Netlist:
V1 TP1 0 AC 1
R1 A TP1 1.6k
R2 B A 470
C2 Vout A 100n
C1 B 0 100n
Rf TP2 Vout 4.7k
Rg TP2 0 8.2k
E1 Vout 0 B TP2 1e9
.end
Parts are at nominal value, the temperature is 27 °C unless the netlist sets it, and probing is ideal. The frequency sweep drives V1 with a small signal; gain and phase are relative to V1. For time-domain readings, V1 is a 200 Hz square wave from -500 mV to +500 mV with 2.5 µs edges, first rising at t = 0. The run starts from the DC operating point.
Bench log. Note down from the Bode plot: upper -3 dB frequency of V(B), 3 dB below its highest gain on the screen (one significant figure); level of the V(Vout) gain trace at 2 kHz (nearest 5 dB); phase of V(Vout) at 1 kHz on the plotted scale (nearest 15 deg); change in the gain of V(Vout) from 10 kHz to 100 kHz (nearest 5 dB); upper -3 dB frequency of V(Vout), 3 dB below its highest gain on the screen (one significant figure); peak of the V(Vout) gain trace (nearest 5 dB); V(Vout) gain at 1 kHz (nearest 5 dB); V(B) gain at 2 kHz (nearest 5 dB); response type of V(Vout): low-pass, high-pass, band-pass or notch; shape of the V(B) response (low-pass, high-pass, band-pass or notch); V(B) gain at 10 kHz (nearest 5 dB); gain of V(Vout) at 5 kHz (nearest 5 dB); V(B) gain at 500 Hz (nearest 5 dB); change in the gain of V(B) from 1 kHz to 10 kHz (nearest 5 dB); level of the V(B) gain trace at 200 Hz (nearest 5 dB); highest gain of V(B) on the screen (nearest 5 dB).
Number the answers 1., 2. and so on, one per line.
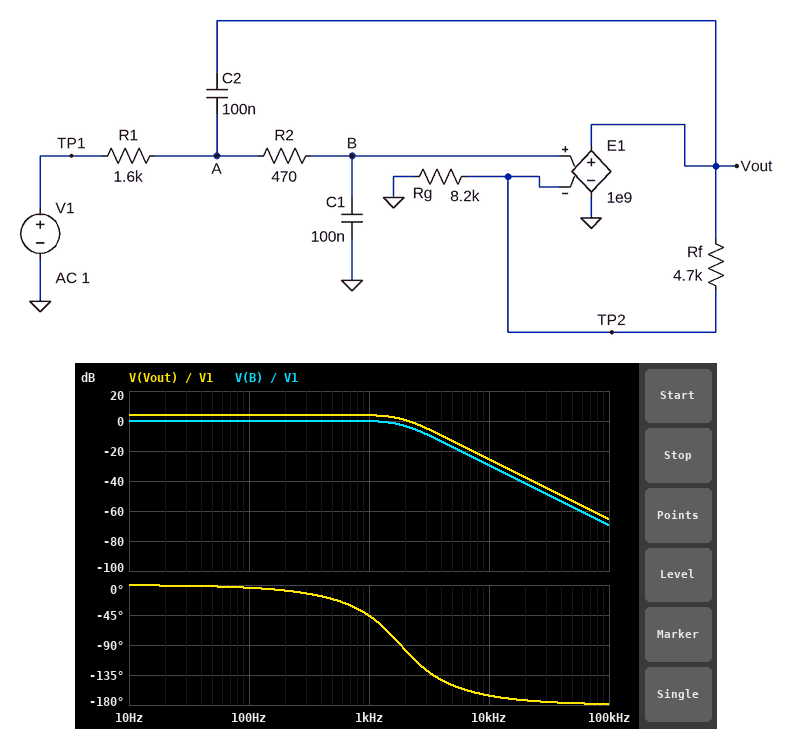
1. 2 kHz
2. 0 dB
3. -45 deg
4. -40 dB
5. 2 kHz
6. 5 dB
7. 5 dB
8. -5 dB
9. low-pass
10. low-pass
11. -30 dB
12. -15 dB
13. 0 dB
14. -30 dB
15. 0 dB
16. 0 dB
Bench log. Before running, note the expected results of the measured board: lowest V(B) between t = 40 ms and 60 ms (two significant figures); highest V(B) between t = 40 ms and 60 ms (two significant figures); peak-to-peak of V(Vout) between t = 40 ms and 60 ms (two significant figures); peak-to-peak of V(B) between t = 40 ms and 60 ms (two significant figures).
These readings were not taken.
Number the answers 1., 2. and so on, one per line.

1. -560 mV
2. 560 mV
3. 1.8 V
4. 1.1 V
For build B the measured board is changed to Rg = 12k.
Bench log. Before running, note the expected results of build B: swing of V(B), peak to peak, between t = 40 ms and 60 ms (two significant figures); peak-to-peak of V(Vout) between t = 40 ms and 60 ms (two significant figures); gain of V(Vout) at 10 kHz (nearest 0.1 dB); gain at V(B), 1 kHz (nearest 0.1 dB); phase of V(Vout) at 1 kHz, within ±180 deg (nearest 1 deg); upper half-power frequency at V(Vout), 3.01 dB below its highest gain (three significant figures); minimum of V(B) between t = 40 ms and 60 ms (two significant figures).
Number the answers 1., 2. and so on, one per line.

1. 1.0 V
2. 1.4 V
3. -26.7 dB
4. -1.2 dB
5. -52 deg
6. 1.52 kHz
7. -510 mV
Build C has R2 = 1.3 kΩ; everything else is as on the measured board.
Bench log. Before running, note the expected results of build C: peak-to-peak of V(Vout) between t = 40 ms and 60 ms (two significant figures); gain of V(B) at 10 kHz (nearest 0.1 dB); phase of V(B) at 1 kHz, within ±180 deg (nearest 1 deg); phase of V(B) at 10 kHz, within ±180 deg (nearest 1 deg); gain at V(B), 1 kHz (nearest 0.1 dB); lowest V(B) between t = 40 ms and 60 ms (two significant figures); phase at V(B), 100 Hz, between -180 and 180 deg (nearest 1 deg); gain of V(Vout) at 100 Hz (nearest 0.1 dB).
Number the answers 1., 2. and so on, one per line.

1. 1.7 V
2. -38.3 dB
3. -82 deg
4. -171 deg
5. -2.0 dB
6. -550 mV
7. -7 deg
8. 3.9 dB
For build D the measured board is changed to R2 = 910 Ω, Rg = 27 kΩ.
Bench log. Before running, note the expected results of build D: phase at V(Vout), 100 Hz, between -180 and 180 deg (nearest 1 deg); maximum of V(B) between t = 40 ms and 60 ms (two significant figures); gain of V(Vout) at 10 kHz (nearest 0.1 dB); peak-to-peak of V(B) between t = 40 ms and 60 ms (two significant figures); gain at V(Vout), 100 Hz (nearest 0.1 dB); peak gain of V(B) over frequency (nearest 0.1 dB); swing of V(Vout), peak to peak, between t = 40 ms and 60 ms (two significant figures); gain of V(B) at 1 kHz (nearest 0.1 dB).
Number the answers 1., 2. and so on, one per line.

1. -8 deg
2. 500 mV
3. -33.9 dB
4. 1.0 V
5. 1.4 dB
6. 0 dB
7. 1.2 V
8. -3.3 dB
